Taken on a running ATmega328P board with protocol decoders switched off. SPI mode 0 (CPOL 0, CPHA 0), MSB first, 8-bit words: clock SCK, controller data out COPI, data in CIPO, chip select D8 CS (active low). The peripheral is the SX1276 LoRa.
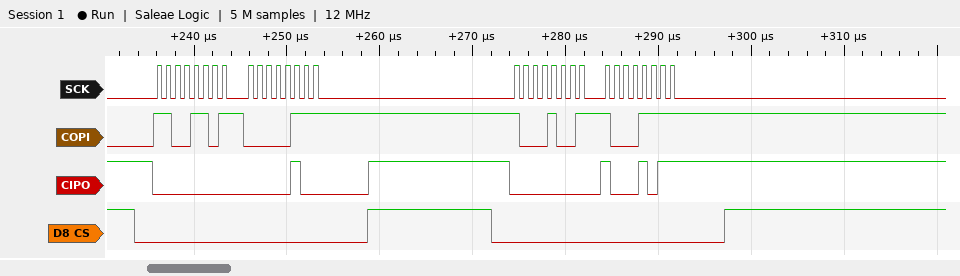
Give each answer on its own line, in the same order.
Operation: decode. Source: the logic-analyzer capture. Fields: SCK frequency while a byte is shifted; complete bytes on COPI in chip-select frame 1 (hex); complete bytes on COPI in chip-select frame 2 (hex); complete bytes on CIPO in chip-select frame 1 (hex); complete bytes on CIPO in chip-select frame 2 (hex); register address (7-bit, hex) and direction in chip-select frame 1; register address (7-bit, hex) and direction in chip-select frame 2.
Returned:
1 MHz
CD 07
89 8F
00 04
00 8B
0x4D write
0x09 write
